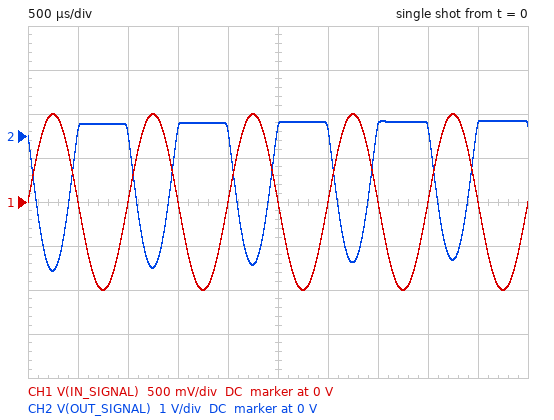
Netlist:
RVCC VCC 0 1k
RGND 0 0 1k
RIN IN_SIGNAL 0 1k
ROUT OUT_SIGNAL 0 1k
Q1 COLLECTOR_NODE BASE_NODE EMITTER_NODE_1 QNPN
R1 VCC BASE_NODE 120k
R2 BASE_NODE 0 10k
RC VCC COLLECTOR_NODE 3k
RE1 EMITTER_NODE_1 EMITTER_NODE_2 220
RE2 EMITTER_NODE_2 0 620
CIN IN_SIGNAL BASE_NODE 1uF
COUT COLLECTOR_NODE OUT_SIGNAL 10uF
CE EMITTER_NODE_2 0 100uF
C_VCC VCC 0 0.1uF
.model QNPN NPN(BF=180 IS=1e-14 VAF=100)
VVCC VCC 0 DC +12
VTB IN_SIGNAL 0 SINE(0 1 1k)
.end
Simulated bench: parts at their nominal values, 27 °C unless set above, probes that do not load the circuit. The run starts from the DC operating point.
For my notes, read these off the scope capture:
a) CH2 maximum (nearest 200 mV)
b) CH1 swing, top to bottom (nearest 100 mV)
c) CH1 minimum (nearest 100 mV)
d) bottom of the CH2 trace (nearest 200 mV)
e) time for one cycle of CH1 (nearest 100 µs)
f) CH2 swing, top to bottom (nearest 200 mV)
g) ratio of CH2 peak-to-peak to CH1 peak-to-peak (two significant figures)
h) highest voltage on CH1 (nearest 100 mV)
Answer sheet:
400 mV
2.0 V
-1.0 V
-3.0 V
1.0 ms
3.4 V
1.7
1.0 V
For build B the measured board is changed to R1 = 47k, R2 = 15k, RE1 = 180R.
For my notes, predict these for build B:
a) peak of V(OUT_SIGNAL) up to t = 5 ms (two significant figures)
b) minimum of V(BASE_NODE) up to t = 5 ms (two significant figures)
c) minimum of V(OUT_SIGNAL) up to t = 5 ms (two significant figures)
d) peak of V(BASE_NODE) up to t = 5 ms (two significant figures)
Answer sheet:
1.9 V
1.3 V
-1.9 V
3.5 V
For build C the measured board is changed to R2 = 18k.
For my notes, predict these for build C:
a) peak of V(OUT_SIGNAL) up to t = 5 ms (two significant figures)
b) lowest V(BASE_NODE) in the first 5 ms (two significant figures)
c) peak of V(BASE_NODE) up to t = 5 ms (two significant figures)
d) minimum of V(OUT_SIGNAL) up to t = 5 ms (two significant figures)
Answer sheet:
820 mV
460 mV
2.5 V
-3.2 V
